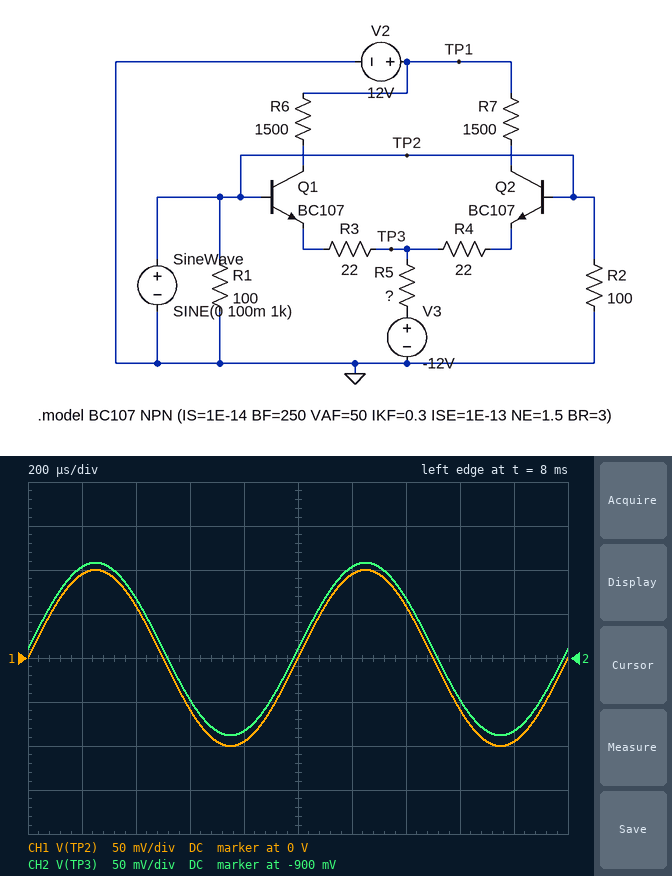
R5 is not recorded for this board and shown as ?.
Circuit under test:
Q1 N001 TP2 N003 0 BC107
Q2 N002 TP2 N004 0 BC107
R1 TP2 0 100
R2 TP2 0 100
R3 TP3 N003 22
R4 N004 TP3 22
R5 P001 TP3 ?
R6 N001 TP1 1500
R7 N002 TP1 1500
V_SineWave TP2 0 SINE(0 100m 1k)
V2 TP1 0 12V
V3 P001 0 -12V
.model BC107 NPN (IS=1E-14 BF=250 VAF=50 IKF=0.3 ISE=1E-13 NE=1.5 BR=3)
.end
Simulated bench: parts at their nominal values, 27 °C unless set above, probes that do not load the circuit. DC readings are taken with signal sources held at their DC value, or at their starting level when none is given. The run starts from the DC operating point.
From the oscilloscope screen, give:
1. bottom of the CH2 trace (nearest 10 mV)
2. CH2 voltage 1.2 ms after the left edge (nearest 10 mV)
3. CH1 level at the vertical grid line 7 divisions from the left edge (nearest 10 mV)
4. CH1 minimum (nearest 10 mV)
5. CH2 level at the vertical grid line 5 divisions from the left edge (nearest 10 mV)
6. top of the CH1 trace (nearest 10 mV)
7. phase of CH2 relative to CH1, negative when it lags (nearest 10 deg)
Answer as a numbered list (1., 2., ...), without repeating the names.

1. -990 mV
2. -800 mV
3. 60 mV
4. -100 mV
5. -890 mV
6. 100 mV
7. 0 deg
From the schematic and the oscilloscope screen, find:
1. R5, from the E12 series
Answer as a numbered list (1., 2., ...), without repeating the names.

1. 680 Ω
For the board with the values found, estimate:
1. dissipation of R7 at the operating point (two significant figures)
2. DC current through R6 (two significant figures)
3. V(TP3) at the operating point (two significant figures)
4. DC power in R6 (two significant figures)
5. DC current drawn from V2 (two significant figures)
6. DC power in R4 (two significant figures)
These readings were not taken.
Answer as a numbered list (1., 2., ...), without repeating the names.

1. 99 mW
2. 8.1 mA
3. -890 mV
4. 99 mW
5. 16 mA
6. 1.5 mW
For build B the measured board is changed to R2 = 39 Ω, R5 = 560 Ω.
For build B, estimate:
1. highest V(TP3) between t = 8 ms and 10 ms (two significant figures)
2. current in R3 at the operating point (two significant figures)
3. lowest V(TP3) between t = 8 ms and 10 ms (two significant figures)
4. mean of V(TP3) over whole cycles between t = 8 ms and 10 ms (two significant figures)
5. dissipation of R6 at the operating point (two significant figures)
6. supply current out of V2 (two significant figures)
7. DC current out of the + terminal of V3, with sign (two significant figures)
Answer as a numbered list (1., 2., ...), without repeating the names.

1. -840 mV
2. 9.9 mA
3. -1.0 V
4. -940 mV
5. 110 mW
6. 17 mA
7. -20 mA
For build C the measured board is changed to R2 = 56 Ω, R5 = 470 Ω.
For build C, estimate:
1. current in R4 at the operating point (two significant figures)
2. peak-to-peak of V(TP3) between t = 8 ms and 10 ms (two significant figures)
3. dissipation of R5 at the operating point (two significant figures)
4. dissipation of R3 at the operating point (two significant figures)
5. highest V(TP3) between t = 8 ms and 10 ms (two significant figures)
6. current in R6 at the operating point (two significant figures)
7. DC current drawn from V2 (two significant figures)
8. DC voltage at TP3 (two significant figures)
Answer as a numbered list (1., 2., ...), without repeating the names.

1. 12 mA
2. 190 mV
3. 260 mW
4. 3.0 mW
5. -900 mV
6. 8.5 mA
7. 17 mA
8. -990 mV
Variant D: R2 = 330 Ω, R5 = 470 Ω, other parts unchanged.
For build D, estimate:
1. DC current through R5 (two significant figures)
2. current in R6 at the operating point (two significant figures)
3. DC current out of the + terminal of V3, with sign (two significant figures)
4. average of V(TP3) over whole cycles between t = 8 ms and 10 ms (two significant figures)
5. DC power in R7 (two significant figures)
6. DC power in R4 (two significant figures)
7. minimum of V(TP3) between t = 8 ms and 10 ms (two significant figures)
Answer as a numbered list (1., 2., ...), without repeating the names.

1. 23 mA
2. 8.5 mA
3. -23 mA
4. -990 mV
5. 110 mW
6. 3.0 mW
7. -1.1 V
